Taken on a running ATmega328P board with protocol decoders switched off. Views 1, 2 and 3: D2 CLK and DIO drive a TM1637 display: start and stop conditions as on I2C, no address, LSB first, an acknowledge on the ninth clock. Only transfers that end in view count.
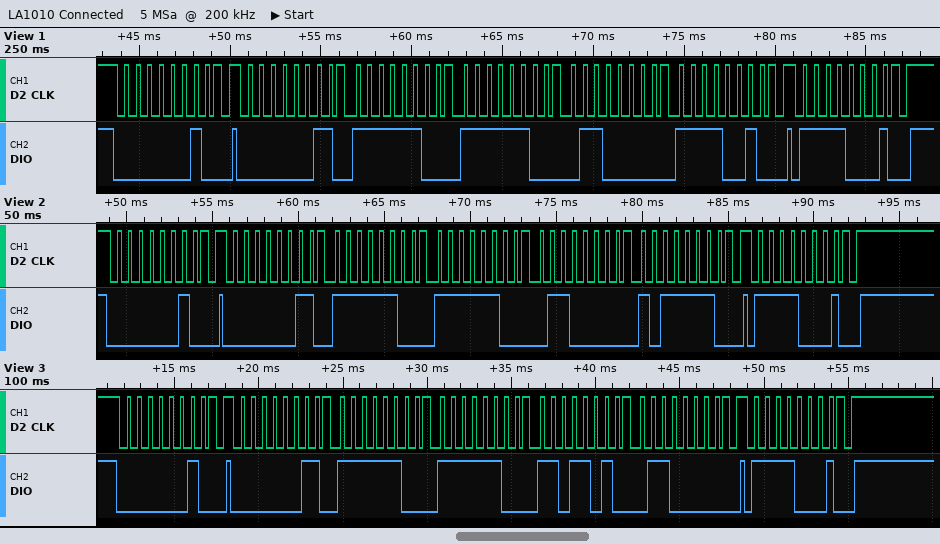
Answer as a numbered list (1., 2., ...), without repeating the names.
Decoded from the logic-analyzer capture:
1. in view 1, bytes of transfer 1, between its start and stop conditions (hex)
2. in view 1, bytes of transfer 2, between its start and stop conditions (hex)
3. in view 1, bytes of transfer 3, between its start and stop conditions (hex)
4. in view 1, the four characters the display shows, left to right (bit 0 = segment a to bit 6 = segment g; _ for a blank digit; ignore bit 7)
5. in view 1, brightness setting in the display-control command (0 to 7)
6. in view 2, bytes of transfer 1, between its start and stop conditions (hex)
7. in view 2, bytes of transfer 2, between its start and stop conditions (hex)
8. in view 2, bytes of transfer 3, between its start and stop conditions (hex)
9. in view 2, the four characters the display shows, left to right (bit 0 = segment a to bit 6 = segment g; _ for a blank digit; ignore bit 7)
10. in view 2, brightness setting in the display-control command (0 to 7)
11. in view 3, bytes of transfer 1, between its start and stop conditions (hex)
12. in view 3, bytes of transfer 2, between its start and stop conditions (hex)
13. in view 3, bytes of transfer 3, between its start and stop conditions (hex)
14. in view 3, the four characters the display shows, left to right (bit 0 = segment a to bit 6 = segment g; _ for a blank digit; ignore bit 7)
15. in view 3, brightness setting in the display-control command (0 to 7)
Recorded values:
1. 40
2. C0 3F 3F 06 4F
3. 8F
4. 0013
5. 7
6. 40
7. C0 3F 3F 06 7D
8. 8F
9. 0016
10. 7
11. 40
12. C0 3F 3F 5B 06
13. 8F
14. 0021
15. 7
